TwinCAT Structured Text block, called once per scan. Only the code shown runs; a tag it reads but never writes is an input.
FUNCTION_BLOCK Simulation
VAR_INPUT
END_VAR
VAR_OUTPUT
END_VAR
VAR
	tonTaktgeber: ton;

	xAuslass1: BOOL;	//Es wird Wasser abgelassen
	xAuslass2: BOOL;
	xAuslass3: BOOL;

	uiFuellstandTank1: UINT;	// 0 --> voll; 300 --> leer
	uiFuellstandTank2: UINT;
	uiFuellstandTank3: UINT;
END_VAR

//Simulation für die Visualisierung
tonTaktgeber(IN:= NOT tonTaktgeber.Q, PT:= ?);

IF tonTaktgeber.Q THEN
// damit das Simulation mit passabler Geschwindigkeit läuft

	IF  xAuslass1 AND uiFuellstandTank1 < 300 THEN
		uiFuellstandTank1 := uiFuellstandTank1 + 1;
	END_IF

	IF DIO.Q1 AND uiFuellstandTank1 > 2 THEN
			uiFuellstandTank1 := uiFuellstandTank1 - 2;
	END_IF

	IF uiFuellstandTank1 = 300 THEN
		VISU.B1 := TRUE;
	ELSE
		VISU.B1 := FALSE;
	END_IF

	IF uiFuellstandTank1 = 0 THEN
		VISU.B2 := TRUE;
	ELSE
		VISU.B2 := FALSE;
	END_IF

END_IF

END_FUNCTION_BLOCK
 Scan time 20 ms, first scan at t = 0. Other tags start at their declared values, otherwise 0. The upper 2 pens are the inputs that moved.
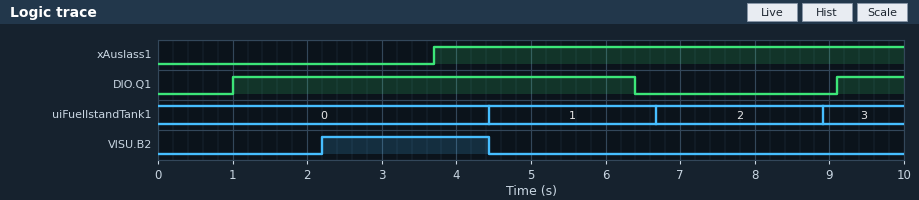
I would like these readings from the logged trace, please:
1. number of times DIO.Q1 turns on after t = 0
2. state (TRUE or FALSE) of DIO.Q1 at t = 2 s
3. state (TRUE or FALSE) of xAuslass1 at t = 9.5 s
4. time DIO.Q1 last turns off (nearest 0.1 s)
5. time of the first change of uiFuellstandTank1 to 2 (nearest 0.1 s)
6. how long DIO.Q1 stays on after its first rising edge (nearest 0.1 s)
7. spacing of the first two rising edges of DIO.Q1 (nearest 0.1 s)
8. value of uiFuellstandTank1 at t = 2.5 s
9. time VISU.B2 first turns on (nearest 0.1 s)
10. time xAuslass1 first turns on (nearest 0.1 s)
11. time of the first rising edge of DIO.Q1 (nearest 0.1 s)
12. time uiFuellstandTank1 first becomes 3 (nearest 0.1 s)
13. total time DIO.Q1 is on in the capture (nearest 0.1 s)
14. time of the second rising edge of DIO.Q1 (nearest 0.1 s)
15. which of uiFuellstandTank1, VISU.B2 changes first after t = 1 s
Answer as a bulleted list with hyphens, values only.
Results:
- 2
- TRUE
- TRUE
- 6.4 s
- 6.7 s
- 5.4 s
- 8.1 s
- 0
- 2.2 s
- 3.7 s
- 1.0 s
- 8.9 s
- 6.3 s
- 9.1 s
- VISU.B2
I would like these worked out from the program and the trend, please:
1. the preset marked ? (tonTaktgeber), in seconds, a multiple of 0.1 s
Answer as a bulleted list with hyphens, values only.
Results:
- 2.2 s
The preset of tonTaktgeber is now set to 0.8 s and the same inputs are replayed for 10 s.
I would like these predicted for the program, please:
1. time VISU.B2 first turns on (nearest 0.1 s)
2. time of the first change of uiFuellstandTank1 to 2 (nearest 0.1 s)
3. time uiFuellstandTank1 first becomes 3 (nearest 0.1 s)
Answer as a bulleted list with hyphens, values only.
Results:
- 0.8 s
- 5.0 s
- 7.5 s
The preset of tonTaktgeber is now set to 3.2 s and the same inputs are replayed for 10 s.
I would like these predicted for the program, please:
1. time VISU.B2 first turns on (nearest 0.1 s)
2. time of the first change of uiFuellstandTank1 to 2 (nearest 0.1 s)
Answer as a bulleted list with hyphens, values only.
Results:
- 3.2 s
- 9.7 s
